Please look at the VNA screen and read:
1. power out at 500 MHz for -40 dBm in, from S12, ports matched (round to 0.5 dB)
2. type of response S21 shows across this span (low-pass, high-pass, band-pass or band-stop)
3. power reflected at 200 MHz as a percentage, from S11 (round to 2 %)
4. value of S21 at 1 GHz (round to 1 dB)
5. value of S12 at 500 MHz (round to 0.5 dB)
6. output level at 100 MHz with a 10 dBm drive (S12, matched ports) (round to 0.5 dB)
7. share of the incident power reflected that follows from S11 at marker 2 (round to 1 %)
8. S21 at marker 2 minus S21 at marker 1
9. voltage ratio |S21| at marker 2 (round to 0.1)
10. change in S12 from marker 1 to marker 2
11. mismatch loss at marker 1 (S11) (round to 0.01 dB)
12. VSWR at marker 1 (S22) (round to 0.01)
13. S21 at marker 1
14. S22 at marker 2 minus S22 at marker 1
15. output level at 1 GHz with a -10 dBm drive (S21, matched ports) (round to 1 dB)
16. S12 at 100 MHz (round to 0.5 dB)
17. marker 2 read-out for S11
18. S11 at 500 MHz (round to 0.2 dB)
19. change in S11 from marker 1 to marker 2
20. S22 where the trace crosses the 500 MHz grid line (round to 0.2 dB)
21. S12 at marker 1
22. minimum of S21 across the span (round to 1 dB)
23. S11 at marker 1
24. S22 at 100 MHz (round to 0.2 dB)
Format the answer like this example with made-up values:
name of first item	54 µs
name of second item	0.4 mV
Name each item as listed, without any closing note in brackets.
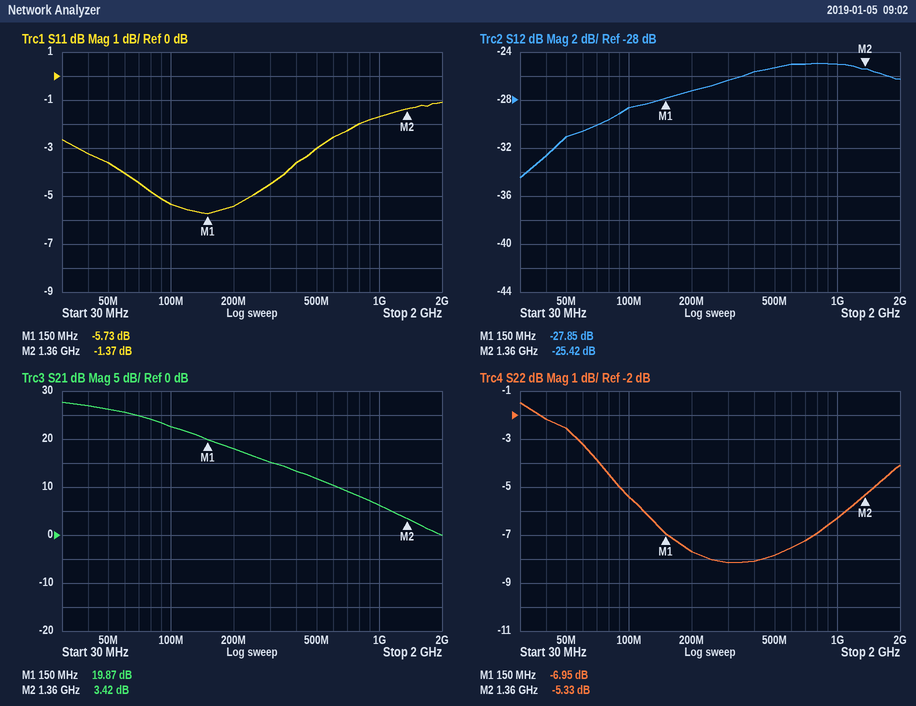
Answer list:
power out at 500 MHz for -40 dBm in, from S12, ports matched	-65.5 dBm
type of response S21 shows across this span	low-pass
power reflected at 200 MHz as a percentage, from S11	28 %
value of S21 at 1 GHz	6 dB
value of S12 at 500 MHz	-25.5 dB
output level at 100 MHz with a 10 dBm drive (S12, matched ports)	-18.5 dBm
share of the incident power reflected that follows from S11 at marker 2	73 %
S21 at marker 2 minus S21 at marker 1	-16.45 dB
voltage ratio |S21| at marker 2	1.5
change in S12 from marker 1 to marker 2	2.43 dB
mismatch loss at marker 1 (S11)	1.35 dB
VSWR at marker 1 (S22)	2.63
S21 at marker 1	19.87 dB
S22 at marker 2 minus S22 at marker 1	1.62 dB
output level at 1 GHz with a -10 dBm drive (S21, matched ports)	-4 dBm
S12 at 100 MHz	-28.5 dB
marker 2 read-out for S11	-1.37 dB
S11 at 500 MHz	-3.0 dB
change in S11 from marker 1 to marker 2	4.36 dB
S22 where the trace crosses the 500 MHz grid line	-7.8 dB
S12 at marker 1	-27.85 dB
minimum of S21 across the span	0 dB
S11 at marker 1	-5.73 dB
S22 at 100 MHz	-5.4 dB
